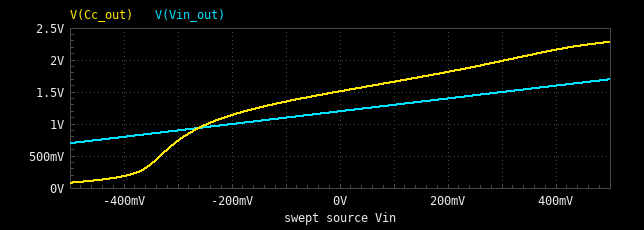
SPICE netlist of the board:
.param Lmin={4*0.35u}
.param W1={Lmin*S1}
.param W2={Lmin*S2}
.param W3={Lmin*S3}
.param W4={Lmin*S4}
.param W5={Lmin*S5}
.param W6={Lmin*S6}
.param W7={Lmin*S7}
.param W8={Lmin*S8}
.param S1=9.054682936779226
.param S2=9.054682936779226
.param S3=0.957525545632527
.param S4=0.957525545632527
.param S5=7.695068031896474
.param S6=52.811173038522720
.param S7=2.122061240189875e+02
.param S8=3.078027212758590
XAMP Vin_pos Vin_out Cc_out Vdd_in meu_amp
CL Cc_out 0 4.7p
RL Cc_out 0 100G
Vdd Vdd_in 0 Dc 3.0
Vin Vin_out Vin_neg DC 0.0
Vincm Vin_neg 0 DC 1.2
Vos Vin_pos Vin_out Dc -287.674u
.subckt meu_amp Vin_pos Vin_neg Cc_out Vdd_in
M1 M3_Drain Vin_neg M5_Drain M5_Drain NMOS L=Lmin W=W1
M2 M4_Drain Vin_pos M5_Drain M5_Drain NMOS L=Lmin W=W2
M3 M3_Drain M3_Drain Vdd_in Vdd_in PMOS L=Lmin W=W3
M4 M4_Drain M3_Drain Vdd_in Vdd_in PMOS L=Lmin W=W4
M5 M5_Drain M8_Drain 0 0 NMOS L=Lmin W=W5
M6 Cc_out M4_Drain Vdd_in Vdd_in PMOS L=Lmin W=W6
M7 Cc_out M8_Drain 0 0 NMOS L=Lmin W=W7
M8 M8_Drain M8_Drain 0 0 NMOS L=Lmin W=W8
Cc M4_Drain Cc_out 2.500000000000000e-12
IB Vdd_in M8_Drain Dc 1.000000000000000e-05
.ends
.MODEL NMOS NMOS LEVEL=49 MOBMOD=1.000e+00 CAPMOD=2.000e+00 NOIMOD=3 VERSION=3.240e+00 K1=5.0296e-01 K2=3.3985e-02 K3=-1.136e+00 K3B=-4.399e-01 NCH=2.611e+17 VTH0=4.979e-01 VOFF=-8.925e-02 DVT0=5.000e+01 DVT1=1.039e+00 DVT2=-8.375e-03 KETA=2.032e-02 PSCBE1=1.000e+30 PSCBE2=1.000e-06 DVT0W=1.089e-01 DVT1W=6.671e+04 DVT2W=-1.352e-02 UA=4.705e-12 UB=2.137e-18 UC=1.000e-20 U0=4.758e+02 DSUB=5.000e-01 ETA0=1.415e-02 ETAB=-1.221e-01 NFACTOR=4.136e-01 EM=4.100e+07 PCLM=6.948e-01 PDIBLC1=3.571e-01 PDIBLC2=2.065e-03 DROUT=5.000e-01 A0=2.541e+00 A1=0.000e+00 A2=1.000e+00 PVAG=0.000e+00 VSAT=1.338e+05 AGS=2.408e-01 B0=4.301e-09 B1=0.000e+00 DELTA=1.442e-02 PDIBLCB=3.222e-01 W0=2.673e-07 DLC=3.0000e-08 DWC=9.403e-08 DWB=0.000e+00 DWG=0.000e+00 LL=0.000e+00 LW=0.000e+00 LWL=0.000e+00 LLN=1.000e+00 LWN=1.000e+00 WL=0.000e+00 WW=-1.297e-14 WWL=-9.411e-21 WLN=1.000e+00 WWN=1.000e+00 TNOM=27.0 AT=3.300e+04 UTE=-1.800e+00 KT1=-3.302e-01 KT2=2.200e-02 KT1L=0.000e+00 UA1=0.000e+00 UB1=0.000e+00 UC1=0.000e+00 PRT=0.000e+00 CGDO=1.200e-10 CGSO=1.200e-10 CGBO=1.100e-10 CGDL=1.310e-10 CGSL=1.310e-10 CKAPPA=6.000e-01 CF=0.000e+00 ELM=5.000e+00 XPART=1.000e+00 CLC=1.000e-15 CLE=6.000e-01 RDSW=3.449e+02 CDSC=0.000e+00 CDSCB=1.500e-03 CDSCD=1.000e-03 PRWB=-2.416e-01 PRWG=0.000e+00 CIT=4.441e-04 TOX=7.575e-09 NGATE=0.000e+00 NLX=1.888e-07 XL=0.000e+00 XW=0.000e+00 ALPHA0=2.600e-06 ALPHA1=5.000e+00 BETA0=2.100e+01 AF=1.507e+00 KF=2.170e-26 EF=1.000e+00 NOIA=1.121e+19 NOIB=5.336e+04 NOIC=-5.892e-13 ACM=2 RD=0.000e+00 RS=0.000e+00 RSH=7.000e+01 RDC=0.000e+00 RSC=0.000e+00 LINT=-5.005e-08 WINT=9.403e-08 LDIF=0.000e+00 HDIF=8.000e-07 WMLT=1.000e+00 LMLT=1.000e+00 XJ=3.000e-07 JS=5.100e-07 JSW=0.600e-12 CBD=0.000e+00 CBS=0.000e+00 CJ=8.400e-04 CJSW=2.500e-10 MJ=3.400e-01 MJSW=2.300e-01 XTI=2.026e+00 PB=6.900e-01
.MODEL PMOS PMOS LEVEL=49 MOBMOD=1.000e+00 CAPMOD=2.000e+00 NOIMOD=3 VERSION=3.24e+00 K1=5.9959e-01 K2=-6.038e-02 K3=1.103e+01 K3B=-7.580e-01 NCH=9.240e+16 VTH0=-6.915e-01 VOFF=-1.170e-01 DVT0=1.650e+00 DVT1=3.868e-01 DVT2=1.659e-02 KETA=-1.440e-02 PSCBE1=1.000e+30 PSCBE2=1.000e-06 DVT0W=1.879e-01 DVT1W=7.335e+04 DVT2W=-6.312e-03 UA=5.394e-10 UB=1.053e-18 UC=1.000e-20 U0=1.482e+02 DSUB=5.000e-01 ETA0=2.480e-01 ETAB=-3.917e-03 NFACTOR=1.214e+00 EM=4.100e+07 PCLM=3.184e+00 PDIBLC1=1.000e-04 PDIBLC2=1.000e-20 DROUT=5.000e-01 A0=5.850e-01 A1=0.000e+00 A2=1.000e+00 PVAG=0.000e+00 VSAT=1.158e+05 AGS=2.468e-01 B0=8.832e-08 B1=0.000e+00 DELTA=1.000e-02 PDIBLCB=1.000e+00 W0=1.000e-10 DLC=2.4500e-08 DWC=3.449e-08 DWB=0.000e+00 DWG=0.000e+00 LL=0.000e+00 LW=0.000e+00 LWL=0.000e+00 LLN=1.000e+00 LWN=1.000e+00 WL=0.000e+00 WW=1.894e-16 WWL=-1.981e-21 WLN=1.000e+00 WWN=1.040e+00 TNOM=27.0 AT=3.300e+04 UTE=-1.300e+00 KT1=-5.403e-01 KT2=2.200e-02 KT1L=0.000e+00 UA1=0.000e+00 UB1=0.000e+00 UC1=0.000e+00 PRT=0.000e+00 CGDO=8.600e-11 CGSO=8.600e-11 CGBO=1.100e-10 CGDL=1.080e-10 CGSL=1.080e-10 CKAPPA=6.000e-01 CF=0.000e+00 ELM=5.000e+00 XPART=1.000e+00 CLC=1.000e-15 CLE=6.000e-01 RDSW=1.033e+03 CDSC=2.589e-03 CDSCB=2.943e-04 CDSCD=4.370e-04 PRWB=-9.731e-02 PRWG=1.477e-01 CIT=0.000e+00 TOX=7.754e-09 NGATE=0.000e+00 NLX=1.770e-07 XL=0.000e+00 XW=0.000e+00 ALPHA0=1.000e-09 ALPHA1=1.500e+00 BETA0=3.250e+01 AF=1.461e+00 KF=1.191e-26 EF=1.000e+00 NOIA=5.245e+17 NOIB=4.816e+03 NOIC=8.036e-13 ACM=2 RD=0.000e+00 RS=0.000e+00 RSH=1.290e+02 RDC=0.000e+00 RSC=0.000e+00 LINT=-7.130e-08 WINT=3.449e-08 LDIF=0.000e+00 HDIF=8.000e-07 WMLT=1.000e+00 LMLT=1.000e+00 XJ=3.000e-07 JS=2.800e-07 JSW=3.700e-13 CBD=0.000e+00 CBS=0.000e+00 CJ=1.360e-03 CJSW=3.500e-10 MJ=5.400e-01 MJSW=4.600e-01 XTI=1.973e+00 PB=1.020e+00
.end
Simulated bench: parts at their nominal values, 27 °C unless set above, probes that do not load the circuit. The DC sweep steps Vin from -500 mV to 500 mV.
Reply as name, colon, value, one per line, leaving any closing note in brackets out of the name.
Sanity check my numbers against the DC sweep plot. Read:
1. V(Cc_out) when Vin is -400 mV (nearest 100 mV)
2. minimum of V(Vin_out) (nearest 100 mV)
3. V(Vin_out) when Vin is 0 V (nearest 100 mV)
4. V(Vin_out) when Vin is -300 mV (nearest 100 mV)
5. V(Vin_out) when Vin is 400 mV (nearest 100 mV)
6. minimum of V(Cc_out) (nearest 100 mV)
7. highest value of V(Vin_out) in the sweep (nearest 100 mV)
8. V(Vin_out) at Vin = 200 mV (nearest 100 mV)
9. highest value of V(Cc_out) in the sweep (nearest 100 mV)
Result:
V(Cc_out) when Vin is -400 mV: 200 mV
minimum of V(Vin_out): 700 mV
V(Vin_out) when Vin is 0 V: 1.2 V
V(Vin_out) when Vin is -300 mV: 900 mV
V(Vin_out) when Vin is 400 mV: 1.6 V
minimum of V(Cc_out): 100 mV
highest value of V(Vin_out) in the sweep: 1.7 V
V(Vin_out) at Vin = 200 mV: 1.4 V
highest value of V(Cc_out) in the sweep: 2.3 V
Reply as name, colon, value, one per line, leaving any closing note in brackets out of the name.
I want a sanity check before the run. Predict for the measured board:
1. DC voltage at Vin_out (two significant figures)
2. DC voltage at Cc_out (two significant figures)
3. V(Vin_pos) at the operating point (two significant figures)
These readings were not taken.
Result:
DC voltage at Vin_out: 1.2 V
DC voltage at Cc_out: 1.5 V
V(Vin_pos) at the operating point: 1.2 V
